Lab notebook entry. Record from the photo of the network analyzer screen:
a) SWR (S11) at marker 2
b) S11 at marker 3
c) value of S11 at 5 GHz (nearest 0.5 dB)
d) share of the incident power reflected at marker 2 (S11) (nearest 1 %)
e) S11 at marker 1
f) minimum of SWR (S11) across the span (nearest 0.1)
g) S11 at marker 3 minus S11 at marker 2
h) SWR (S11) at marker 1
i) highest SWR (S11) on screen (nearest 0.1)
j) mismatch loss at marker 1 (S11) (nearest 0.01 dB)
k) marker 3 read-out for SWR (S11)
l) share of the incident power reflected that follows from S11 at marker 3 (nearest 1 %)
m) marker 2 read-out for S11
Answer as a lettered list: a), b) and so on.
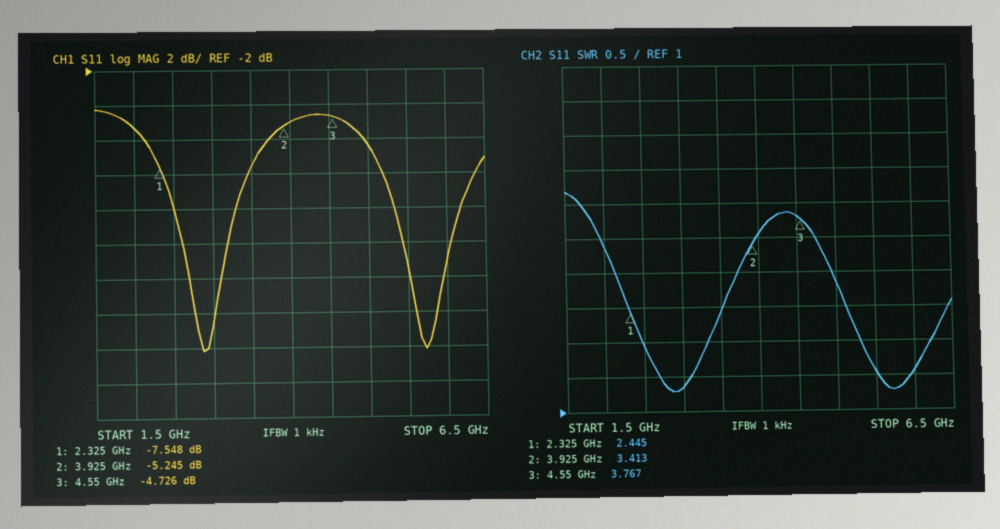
a) 3.413
b) -4.726 dB
c) -6.5 dB
d) 30 %
e) -7.548 dB
f) 1.3
g) 0.519 dB
h) 2.445
i) 4.2
j) 0.84 dB
k) 3.767
l) 34 %
m) -5.245 dB
